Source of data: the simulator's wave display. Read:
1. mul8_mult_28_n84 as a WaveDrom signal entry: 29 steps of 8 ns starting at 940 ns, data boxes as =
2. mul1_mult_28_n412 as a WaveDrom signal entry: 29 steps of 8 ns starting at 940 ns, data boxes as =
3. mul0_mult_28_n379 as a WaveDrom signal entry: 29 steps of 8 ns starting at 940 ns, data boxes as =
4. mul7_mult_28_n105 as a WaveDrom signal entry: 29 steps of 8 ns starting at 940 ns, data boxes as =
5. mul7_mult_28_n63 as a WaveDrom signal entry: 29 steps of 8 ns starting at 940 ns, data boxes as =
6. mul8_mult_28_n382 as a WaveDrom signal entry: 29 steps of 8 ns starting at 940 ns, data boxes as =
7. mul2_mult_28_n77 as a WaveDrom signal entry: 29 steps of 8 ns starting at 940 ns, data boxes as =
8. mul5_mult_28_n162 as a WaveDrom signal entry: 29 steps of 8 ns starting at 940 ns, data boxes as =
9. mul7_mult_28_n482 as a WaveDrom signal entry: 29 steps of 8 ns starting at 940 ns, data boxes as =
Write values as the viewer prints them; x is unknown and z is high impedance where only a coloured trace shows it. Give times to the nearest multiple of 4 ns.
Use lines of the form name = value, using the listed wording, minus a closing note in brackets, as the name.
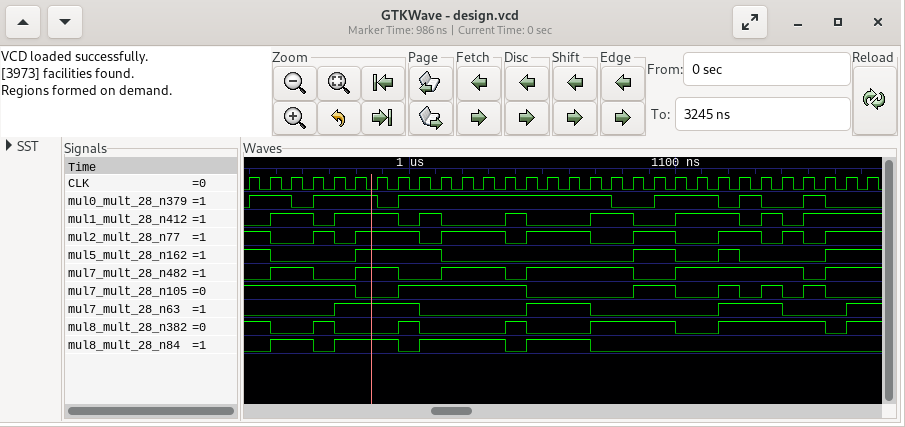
mul8_mult_28_n84 as a WaveDrom signal entry: 29 steps of 8 ns starting at 940 ns, data boxes as = = {name: 'mul8_mult_28_n84', wave: '01.01..01...01..0............'}
mul1_mult_28_n412 as a WaveDrom signal entry: 29 steps of 8 ns starting at 940 ns, data boxes as = = {name: 'mul1_mult_28_n412', wave: '01.01..010..10..1.0.1..0101..'}
mul0_mult_28_n379 as a WaveDrom signal entry: 29 steps of 8 ns starting at 940 ns, data boxes as = = {name: 'mul0_mult_28_n379', wave: '1.01..01.........0.1..010.10.'}
mul7_mult_28_n105 as a WaveDrom signal entry: 29 steps of 8 ns starting at 940 ns, data boxes as = = {name: 'mul7_mult_28_n105', wave: '1....0.1.....0....1.0.101010.'}
mul7_mult_28_n63 as a WaveDrom signal entry: 29 steps of 8 ns starting at 940 ns, data boxes as = = {name: 'mul7_mult_28_n63', wave: '0...1...0....1..0.....1..0..1'}
mul8_mult_28_n382 as a WaveDrom signal entry: 29 steps of 8 ns starting at 940 ns, data boxes as = = {name: 'mul8_mult_28_n382', wave: '10.10..10...10..1...0.1....01'}
mul2_mult_28_n77 as a WaveDrom signal entry: 29 steps of 8 ns starting at 940 ns, data boxes as = = {name: 'mul2_mult_28_n77', wave: '10.101..01..01..0.1.0.1.0101.'}
mul5_mult_28_n162 as a WaveDrom signal entry: 29 steps of 8 ns starting at 940 ns, data boxes as = = {name: 'mul5_mult_28_n162', wave: '10...1...0........1.0.10...1.'}
mul7_mult_28_n482 as a WaveDrom signal entry: 29 steps of 8 ns starting at 940 ns, data boxes as = = {name: 'mul7_mult_28_n482', wave: '01.0.1.0.1..01....0.1.....01.'}
